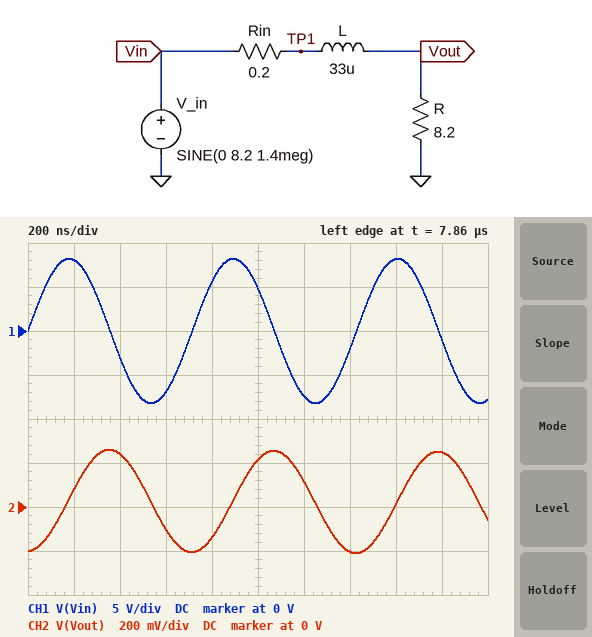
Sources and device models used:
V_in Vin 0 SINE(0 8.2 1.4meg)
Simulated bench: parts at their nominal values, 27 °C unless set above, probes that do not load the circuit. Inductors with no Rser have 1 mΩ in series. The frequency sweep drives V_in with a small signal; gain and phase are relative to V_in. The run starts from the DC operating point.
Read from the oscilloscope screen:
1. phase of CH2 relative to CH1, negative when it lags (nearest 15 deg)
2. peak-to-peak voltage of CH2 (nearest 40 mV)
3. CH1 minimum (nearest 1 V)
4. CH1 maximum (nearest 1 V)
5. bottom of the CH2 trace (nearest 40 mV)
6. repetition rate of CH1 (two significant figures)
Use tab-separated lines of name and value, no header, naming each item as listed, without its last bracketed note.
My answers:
phase of CH2 relative to CH1, negative when it lags	-90 deg
peak-to-peak voltage of CH2	480 mV
CH1 minimum	-8 V
CH1 maximum	8 V
bottom of the CH2 trace	-200 mV
repetition rate of CH1	1.4 MHz
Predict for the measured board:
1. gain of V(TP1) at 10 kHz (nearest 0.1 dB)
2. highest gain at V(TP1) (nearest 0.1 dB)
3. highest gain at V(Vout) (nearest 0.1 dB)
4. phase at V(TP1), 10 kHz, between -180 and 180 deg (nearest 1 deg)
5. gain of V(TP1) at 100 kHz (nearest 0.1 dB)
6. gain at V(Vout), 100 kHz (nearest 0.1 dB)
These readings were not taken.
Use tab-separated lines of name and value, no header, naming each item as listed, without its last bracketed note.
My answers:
gain of V(TP1) at 10 kHz	-0.2 dB
highest gain at V(TP1)	0 dB
highest gain at V(Vout)	-0.2 dB
phase at V(TP1), 10 kHz, between -180 and 180 deg	0 deg
gain of V(TP1) at 100 kHz	0 dB
gain at V(Vout), 100 kHz	-8.7 dB
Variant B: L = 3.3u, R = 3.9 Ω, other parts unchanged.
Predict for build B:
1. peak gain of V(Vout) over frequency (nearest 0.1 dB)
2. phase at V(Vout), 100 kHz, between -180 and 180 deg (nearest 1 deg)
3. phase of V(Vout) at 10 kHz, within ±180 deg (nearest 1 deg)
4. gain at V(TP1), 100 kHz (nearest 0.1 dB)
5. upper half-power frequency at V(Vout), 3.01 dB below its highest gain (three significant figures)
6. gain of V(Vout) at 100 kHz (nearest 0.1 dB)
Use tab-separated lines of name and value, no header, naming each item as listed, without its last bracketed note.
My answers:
peak gain of V(Vout) over frequency	-0.4 dB
phase at V(Vout), 100 kHz, between -180 and 180 deg	-27 deg
phase of V(Vout) at 10 kHz, within ±180 deg	-3 deg
gain at V(TP1), 100 kHz	-0.3 dB
upper half-power frequency at V(Vout), 3.01 dB below its highest gain	198 kHz
gain of V(Vout) at 100 kHz	-1.4 dB
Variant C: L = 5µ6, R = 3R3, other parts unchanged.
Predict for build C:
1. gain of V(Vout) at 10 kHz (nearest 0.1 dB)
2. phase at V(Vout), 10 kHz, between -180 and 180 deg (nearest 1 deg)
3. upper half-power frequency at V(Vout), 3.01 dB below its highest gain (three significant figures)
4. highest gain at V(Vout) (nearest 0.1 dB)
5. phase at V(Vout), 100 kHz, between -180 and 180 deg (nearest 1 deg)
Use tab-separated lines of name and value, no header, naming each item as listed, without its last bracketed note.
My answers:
gain of V(Vout) at 10 kHz	-0.6 dB
phase at V(Vout), 10 kHz, between -180 and 180 deg	-6 deg
upper half-power frequency at V(Vout), 3.01 dB below its highest gain	99.5 kHz
highest gain at V(Vout)	-0.5 dB
phase at V(Vout), 100 kHz, between -180 and 180 deg	-45 deg
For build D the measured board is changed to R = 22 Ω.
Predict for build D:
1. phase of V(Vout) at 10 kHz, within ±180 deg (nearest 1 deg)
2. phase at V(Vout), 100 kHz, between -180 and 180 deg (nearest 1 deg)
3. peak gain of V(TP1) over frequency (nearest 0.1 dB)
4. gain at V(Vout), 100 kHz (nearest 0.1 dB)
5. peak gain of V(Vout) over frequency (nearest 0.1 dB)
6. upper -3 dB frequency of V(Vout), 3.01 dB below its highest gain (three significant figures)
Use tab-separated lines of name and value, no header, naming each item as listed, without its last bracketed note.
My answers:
phase of V(Vout) at 10 kHz, within ±180 deg	-5 deg
phase at V(Vout), 100 kHz, between -180 and 180 deg	-43 deg
peak gain of V(TP1) over frequency	0 dB
gain at V(Vout), 100 kHz	-2.8 dB
peak gain of V(Vout) over frequency	-0.1 dB
upper -3 dB frequency of V(Vout), 3.01 dB below its highest gain	107 kHz
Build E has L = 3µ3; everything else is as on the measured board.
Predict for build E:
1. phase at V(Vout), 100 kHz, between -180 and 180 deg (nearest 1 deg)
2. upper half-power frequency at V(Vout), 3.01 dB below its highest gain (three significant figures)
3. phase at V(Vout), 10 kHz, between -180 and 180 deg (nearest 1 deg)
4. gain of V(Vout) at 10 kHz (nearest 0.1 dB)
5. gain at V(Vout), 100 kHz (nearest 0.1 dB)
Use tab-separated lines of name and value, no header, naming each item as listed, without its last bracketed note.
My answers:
phase at V(Vout), 100 kHz, between -180 and 180 deg	-14 deg
upper half-power frequency at V(Vout), 3.01 dB below its highest gain	405 kHz
phase at V(Vout), 10 kHz, between -180 and 180 deg	-1 deg
gain of V(Vout) at 10 kHz	-0.2 dB
gain at V(Vout), 100 kHz	-0.5 dB
